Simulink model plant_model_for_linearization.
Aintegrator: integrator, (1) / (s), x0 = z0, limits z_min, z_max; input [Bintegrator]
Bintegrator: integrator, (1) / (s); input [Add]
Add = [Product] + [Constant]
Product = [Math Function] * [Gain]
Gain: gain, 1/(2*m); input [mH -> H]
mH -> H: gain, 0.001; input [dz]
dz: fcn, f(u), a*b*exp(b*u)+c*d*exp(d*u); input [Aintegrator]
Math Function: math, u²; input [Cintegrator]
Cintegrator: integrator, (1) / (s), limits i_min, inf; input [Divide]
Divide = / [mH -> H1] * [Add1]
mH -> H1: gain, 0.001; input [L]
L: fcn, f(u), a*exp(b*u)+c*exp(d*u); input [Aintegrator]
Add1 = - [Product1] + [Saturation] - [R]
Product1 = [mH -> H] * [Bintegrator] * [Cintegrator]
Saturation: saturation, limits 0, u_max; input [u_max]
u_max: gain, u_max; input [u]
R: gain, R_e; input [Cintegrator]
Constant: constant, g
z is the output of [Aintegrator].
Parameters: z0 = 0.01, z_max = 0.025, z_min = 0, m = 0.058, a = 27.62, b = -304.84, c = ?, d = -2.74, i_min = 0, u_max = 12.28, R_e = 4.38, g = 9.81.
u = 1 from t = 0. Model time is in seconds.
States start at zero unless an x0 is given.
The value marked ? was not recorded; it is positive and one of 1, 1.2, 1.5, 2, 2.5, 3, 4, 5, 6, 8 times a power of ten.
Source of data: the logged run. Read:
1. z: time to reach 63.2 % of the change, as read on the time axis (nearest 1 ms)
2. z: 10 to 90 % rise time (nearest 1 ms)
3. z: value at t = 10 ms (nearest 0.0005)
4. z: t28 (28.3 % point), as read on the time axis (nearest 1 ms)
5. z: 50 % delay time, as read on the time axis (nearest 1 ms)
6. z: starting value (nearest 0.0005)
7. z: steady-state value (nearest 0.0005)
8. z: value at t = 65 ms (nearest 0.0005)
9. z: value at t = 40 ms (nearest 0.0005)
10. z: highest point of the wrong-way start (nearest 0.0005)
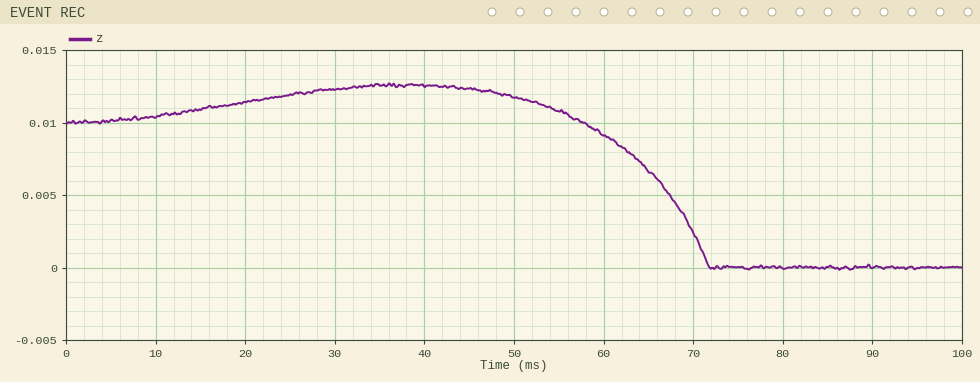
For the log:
69 ms
11 ms
0.0105
64 ms
67 ms
0.0100
0.0000
0.0065
0.0125
0.0125
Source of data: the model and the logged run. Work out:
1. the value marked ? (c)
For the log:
120
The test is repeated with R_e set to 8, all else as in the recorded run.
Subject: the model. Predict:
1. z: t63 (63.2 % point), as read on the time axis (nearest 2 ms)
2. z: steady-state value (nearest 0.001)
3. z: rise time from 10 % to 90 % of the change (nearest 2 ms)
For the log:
62 ms
0.025
58 ms
